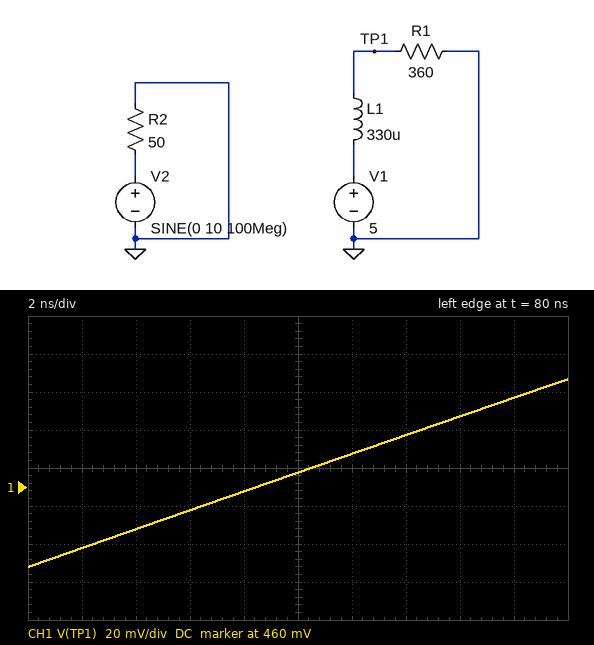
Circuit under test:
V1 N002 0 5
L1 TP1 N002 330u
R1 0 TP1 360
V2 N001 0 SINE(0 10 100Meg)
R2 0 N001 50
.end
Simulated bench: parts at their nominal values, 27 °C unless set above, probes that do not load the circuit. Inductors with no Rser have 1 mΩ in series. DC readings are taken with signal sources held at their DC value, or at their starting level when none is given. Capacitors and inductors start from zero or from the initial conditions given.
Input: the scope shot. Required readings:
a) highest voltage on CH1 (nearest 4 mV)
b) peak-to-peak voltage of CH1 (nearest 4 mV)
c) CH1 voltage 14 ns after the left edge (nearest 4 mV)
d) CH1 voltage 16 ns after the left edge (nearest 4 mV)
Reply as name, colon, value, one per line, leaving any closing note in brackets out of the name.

highest voltage on CH1: 516 mV
peak-to-peak voltage of CH1: 100 mV
CH1 voltage 14 ns after the left edge: 488 mV
CH1 voltage 16 ns after the left edge: 496 mV
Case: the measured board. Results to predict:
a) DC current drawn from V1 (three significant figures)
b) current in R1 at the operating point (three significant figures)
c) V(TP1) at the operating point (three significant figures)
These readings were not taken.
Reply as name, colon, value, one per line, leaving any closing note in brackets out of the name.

DC current drawn from V1: 13.9 mA
current in R1 at the operating point: 13.9 mA
V(TP1) at the operating point: 5.00 V
